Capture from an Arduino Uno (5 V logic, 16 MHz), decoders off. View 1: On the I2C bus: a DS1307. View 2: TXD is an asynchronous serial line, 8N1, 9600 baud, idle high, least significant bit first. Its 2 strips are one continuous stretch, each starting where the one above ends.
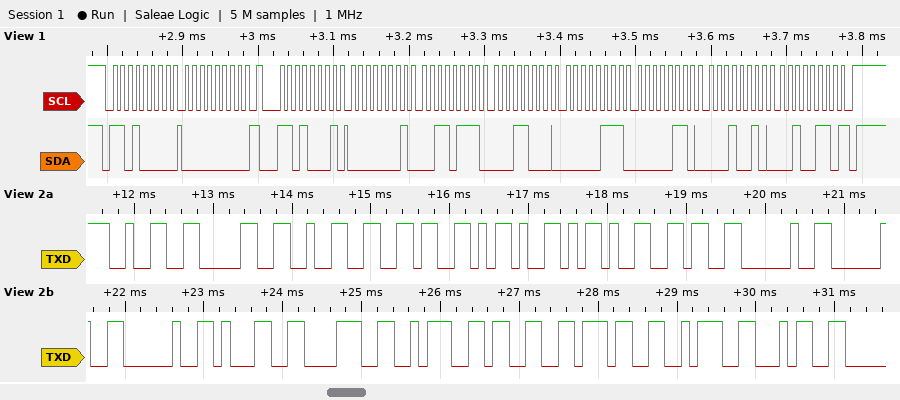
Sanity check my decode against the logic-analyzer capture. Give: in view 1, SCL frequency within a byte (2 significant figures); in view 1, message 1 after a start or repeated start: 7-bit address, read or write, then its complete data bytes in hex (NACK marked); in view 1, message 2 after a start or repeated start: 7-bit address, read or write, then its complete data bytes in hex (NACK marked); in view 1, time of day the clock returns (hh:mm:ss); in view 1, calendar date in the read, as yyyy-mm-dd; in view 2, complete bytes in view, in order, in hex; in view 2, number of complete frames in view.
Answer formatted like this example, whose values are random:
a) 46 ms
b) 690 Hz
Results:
a) 100 kHz
b) 0x68 write: 00
c) 0x68 read: 01 37 18 07 06 12 26 NACK
d) 18:37:01
e) 2026-12-06
f) 32 30 32 36 2D 2D 36 20 20 20 31 38 3A 33 37 3A 34
g) 17
